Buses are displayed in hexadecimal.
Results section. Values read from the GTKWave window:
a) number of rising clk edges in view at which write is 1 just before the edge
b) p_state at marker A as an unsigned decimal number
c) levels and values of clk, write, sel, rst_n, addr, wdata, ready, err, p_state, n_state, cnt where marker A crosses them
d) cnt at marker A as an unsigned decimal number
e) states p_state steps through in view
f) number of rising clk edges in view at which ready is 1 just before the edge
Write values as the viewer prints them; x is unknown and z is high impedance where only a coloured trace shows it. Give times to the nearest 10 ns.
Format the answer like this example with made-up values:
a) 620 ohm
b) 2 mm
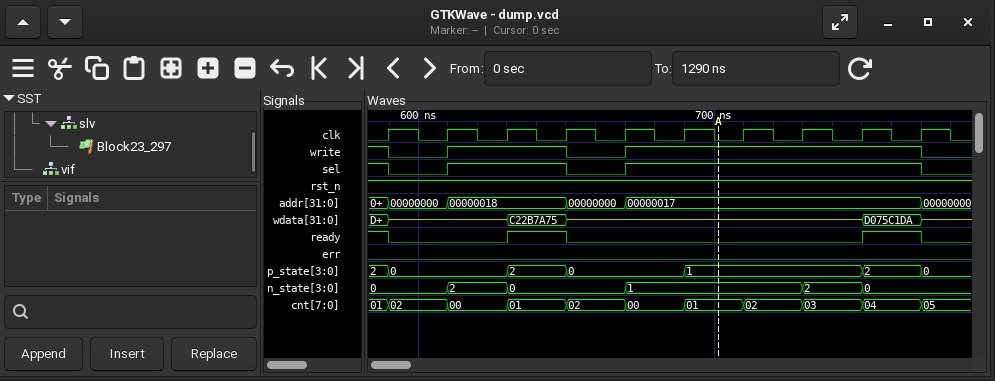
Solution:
a) 8
b) 1
c) clk=0, write=1, sel=1, rst_n=1, addr=00000017, wdata=z, ready=0, err=0, p_state=1, n_state=1, cnt=01
d) 1
e) 2, 0, 2, 0, 1, 2, 0
f) 3
